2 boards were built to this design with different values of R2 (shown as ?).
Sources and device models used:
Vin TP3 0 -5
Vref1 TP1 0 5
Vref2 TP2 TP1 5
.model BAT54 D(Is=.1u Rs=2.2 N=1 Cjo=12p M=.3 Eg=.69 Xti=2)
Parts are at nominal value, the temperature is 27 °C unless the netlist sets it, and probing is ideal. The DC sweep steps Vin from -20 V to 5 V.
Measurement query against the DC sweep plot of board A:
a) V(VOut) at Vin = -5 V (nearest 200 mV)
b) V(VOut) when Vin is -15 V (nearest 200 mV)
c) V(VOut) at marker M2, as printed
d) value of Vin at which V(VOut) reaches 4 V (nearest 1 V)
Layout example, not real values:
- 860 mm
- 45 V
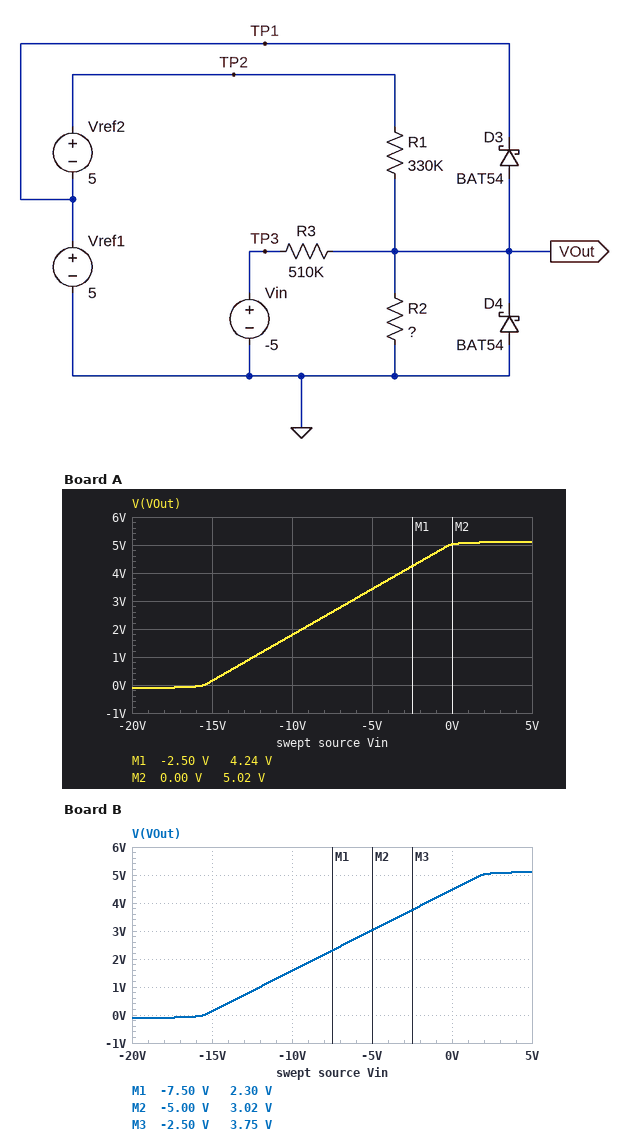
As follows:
- 3.4 V
- 200 mV
- 5.02 V
- -3 V
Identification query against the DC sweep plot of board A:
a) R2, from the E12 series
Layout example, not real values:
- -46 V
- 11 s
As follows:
- 1 MΩ
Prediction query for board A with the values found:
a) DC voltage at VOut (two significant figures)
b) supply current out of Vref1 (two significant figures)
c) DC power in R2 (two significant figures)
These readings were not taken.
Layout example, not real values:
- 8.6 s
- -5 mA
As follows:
- 3.4 V
- 20 µA
- 12 µW
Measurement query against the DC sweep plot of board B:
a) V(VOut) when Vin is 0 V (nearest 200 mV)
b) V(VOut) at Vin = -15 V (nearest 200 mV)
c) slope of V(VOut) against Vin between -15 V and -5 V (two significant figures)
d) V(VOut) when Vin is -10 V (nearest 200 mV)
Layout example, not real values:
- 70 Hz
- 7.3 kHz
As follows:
- 4.4 V
- 200 mV
- 0.29 V/V
- 1.6 V
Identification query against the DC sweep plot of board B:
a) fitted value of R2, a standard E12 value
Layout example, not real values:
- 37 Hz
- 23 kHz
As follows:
- 560 kΩ
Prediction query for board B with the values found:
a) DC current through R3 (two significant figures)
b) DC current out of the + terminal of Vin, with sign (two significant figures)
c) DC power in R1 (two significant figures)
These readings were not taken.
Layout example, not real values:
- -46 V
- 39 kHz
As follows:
- 16 µA
- -16 µA
- 150 µW
